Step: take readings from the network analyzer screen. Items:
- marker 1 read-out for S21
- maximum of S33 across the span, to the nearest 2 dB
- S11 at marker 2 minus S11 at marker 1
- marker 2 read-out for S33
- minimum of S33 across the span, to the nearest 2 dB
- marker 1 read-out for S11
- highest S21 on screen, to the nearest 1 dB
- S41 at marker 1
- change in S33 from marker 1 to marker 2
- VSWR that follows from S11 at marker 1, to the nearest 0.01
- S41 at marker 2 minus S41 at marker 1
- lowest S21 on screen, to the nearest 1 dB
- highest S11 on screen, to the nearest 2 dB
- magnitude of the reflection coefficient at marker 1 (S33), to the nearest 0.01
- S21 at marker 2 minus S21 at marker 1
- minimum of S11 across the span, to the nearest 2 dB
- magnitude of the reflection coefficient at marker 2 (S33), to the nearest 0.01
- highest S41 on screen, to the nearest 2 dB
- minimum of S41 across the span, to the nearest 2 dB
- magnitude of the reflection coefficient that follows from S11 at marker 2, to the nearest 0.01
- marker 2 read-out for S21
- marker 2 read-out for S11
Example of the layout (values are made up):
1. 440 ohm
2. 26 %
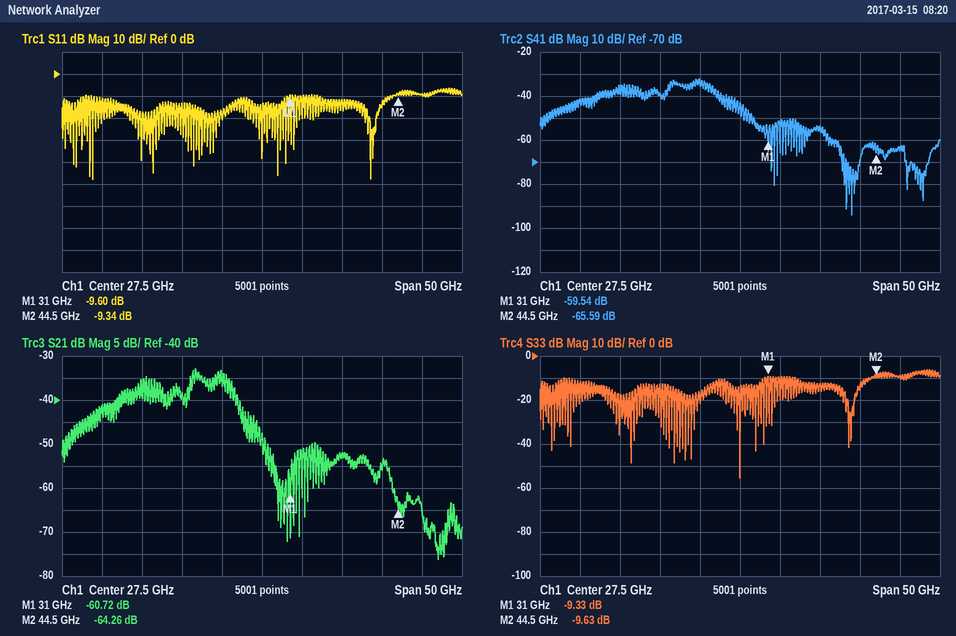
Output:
1. -60.72 dB
2. -6 dB
3. 0.26 dB
4. -9.63 dB
5. -56 dB
6. -9.60 dB
7. -33 dB
8. -59.54 dB
9. -0.30 dB
10. 1.99
11. -6.05 dB
12. -76 dB
13. -6 dB
14. 0.34
15. -3.54 dB
16. -48 dB
17. 0.33
18. -32 dB
19. -94 dB
20. 0.34
21. -64.26 dB
22. -9.34 dB
